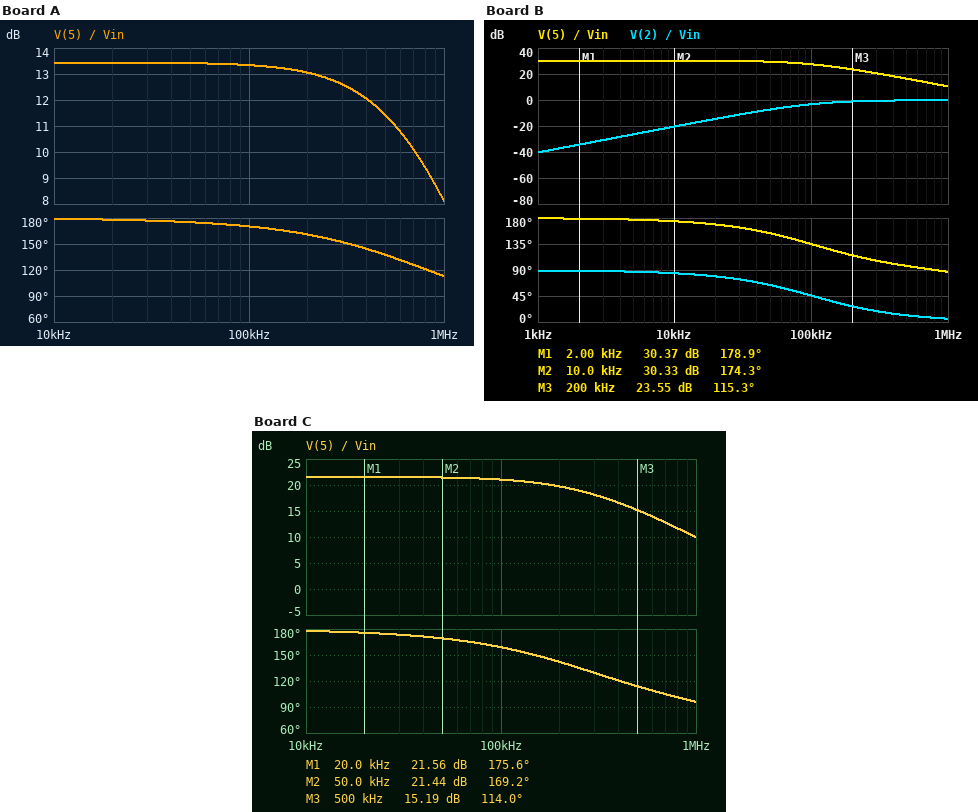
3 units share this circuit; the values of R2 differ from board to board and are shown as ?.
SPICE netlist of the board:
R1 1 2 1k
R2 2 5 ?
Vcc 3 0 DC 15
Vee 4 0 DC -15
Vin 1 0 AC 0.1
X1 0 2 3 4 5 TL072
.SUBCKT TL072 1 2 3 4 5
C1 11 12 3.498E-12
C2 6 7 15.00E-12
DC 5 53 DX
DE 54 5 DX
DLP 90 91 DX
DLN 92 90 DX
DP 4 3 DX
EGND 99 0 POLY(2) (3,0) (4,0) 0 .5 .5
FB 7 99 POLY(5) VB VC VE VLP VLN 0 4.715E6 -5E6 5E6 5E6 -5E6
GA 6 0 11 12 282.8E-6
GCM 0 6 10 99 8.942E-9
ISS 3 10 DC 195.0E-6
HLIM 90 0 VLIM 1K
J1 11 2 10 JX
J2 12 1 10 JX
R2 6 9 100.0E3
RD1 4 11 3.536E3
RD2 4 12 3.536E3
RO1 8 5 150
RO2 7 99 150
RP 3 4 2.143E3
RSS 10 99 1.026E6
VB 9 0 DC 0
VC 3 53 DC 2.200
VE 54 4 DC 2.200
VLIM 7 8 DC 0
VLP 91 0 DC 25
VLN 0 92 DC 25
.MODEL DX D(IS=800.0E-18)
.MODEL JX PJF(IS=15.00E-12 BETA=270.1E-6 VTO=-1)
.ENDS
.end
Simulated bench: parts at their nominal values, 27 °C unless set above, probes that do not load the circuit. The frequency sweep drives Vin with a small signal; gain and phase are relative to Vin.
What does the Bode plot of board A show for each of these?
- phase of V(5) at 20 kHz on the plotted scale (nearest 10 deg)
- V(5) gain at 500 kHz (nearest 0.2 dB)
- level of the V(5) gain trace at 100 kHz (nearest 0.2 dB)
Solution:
180 deg
11.4 dB
13.4 dB
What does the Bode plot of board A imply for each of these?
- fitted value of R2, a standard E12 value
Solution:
4.7 kΩ
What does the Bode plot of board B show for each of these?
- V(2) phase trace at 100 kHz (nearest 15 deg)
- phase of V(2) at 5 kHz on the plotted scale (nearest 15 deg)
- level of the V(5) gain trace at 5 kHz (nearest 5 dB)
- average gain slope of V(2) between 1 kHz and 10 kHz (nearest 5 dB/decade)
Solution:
45 deg
90 deg
30 dB
20 dB/decade
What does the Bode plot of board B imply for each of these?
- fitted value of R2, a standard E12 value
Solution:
33 kΩ
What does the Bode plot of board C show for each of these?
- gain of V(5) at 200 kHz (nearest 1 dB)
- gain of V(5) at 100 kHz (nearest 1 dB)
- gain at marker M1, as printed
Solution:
20 dB
21 dB
21.56 dB
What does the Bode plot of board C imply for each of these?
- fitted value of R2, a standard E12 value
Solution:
12 kΩ
